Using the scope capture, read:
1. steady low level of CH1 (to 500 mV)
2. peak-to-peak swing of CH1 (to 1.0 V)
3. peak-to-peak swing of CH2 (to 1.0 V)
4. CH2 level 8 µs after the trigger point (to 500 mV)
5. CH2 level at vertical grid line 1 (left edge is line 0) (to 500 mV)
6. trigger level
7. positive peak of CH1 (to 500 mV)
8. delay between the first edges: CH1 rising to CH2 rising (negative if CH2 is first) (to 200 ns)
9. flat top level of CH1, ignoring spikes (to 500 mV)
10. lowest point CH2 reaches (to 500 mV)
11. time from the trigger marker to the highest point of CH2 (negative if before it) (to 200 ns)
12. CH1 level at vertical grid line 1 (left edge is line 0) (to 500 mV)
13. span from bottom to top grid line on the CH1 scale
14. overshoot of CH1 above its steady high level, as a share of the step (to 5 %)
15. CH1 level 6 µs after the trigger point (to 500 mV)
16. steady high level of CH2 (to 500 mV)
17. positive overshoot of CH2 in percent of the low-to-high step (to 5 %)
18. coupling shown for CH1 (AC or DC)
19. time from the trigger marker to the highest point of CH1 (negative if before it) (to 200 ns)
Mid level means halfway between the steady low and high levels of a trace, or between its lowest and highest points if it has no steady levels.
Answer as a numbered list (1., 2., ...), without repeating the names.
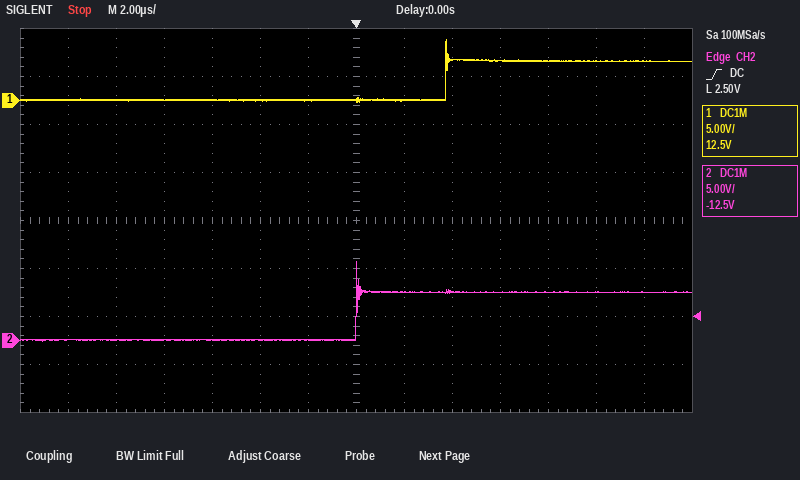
1. 0.0 V
2. 7.0 V
3. 8.0 V
4. 5.0 V
5. 0.0 V
6. 2.50 V
7. 6.5 V
8. -3.8 µs
9. 4.0 V
10. 0.0 V
11. 0.0 µs
12. 0.0 V
13. 40 V
14. 55 %
15. 4.0 V
16. 5.0 V
17. 65 %
18. DC
19. +3.8 µs
